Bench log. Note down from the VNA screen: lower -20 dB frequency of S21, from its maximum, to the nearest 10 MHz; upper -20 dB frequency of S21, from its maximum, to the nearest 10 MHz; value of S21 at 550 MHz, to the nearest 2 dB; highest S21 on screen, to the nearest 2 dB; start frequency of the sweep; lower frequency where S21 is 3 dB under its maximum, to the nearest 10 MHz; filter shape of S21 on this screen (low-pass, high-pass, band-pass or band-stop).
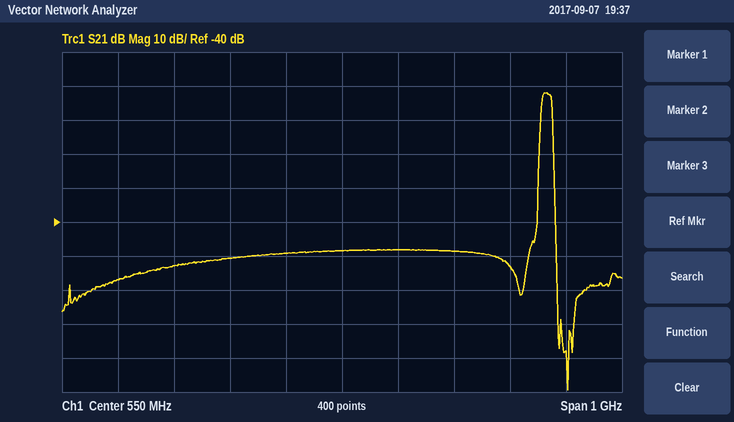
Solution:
900 MHz
930 MHz
-48 dB
-2 dB
50 MHz
910 MHz
band-pass
